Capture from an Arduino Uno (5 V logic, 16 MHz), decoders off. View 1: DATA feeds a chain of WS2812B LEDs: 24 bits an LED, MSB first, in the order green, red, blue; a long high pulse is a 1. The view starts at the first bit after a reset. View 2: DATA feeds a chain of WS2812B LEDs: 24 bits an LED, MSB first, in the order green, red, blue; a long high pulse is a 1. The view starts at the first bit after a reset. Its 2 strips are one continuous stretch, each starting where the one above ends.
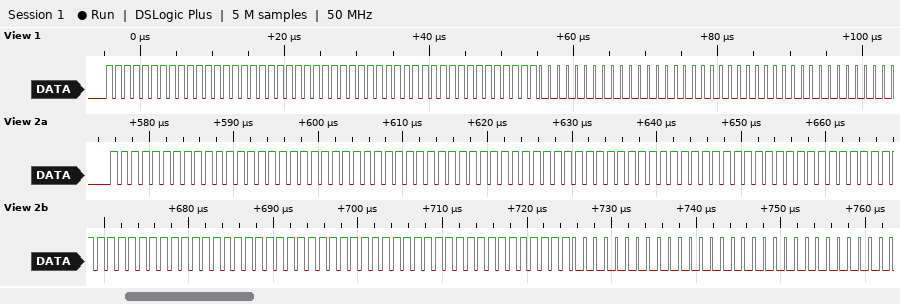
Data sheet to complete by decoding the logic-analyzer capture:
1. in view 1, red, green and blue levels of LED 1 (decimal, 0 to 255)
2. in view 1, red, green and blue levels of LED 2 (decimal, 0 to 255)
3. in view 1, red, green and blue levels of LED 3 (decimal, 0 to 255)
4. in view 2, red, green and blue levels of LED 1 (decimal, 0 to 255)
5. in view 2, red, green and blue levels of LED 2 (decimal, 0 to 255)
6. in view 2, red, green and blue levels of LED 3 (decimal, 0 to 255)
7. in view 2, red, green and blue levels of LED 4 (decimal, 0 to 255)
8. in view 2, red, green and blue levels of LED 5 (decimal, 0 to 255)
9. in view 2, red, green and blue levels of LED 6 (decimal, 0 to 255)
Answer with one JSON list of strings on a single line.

["255, 255, 255", "255, 255, 255", "0, 0, 0", "255, 255, 255", "255, 255, 255", "255, 255, 255", "255, 255, 255", "255, 255, 255", "0, 0, 0"]
